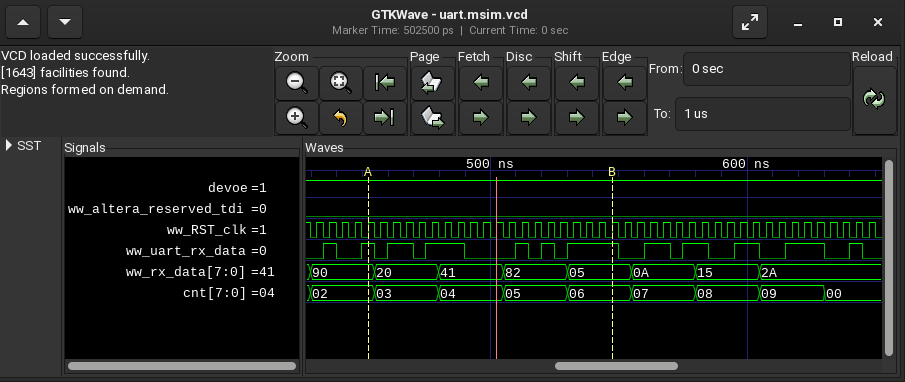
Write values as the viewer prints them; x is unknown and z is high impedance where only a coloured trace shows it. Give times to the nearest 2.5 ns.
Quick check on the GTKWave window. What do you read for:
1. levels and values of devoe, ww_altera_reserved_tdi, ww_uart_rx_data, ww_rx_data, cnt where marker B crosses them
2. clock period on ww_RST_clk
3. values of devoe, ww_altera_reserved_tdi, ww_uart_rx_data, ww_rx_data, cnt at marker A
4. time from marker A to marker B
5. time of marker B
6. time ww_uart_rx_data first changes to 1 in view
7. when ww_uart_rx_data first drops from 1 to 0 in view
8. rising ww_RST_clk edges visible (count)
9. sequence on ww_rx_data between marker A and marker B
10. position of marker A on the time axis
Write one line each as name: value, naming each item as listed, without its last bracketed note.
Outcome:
levels and values of devoe, ww_altera_reserved_tdi, ww_uart_rx_data, ww_rx_data, cnt where marker B crosses them: devoe=1, ww_altera_reserved_tdi=0, ww_uart_rx_data=1, ww_rx_data=05, cnt=06
clock period on ww_RST_clk: 5 ns
values of devoe, ww_altera_reserved_tdi, ww_uart_rx_data, ww_rx_data, cnt at marker A: devoe=1, ww_altera_reserved_tdi=0, ww_uart_rx_data=1, ww_rx_data=90, cnt=02
time from marker A to marker B: 95 ns
time of marker B: 547.5 ns
time ww_uart_rx_data first changes to 1 in view: 435 ns
when ww_uart_rx_data first drops from 1 to 0 in view: 440 ns
rising ww_RST_clk edges visible: 44
sequence on ww_rx_data between marker A and marker B: 90, 20, 41, 82, 05
position of marker A on the time axis: 452.5 ns
